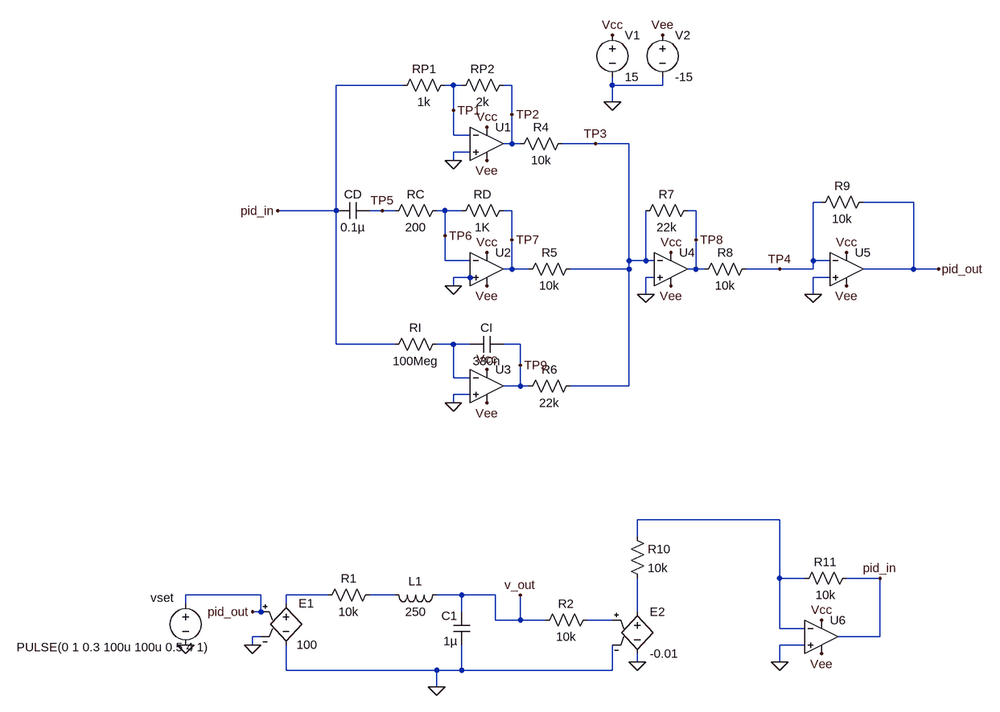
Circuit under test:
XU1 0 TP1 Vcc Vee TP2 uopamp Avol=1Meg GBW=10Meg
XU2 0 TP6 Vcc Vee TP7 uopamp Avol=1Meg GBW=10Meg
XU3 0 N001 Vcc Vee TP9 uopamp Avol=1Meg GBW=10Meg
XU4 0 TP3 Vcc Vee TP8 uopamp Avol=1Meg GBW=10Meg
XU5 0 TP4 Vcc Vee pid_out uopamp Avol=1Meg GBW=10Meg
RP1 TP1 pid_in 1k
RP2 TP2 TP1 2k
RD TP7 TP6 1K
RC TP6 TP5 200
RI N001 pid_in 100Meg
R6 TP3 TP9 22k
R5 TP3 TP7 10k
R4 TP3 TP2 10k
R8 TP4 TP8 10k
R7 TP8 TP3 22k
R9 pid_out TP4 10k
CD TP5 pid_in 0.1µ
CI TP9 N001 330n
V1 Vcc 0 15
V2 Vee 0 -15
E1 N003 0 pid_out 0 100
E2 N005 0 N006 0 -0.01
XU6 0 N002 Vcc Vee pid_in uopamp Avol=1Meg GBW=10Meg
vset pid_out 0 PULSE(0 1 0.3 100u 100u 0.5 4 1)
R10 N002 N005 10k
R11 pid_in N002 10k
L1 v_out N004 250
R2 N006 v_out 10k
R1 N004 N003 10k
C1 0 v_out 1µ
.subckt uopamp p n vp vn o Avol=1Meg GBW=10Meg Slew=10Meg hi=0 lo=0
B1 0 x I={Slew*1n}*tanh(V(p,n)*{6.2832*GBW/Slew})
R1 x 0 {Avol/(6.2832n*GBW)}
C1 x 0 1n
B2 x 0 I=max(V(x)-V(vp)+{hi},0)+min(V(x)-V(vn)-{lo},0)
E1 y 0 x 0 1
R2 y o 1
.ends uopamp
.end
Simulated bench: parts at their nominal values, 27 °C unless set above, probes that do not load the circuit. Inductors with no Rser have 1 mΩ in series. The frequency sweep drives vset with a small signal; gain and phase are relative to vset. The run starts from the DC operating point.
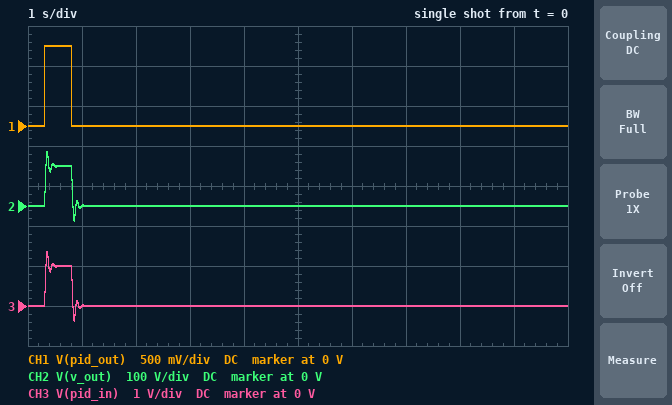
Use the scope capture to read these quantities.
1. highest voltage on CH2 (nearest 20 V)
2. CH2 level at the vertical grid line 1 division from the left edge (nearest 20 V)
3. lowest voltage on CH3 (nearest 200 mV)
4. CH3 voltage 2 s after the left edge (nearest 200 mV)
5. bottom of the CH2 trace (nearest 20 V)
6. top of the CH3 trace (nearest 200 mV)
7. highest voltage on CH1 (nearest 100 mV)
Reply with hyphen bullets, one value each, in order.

- 140 V
- 0 V
- -400 mV
- 0 V
- -40 V
- 1.4 V
- 1.0 V
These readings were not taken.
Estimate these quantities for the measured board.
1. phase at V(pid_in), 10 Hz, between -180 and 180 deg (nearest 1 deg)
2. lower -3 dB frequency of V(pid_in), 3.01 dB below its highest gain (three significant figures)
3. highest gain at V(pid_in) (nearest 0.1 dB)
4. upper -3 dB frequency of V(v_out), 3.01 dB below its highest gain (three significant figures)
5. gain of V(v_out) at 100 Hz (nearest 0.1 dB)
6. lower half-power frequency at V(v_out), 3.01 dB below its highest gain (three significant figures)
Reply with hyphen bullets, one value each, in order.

- -89 deg
- 4.50 Hz
- 4.4 dB
- 11.9 Hz
- 0.2 dB
- 4.50 Hz
